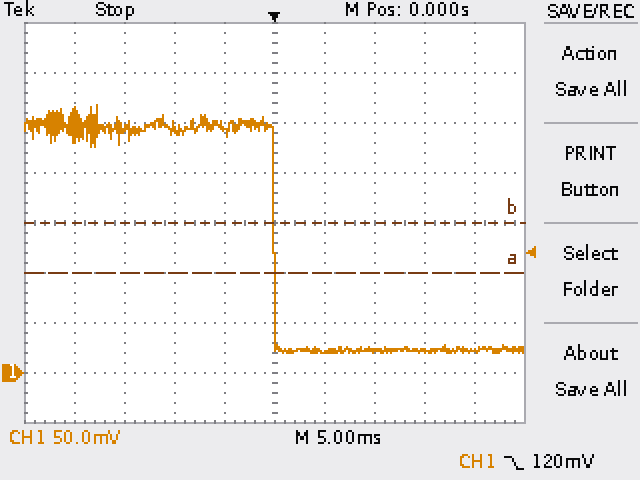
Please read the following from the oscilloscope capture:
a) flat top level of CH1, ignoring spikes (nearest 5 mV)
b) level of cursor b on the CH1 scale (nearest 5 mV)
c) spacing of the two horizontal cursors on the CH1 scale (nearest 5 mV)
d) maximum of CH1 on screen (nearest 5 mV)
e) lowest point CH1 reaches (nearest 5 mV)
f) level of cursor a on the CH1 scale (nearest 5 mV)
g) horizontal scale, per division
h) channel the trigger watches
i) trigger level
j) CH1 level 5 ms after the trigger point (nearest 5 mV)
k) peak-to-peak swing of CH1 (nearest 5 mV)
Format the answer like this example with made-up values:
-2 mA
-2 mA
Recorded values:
245 mV
150 mV
50 mV
270 mV
20 mV
100 mV
5 ms
CH1
120 mV
20 mV
250 mV
